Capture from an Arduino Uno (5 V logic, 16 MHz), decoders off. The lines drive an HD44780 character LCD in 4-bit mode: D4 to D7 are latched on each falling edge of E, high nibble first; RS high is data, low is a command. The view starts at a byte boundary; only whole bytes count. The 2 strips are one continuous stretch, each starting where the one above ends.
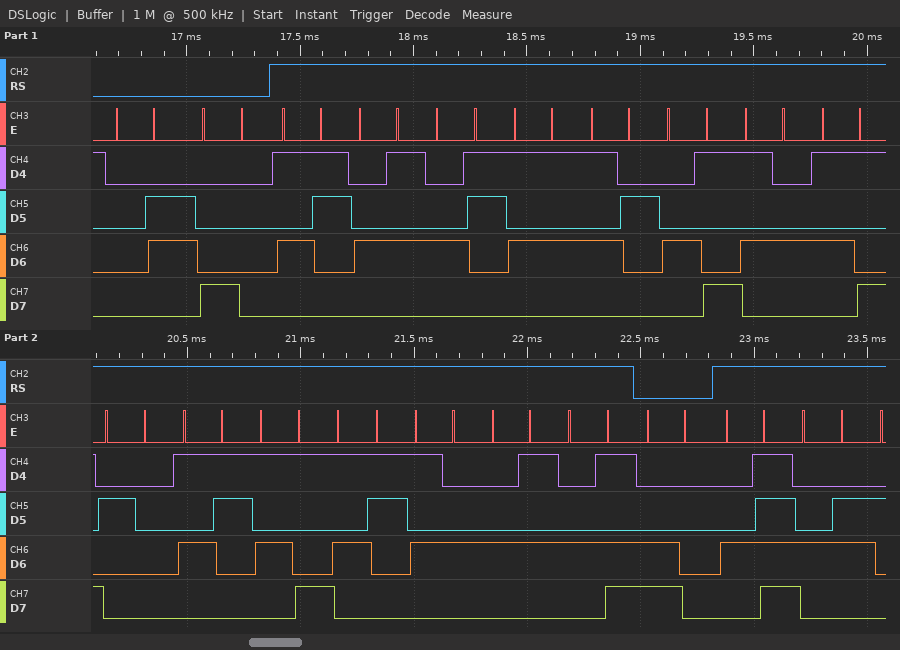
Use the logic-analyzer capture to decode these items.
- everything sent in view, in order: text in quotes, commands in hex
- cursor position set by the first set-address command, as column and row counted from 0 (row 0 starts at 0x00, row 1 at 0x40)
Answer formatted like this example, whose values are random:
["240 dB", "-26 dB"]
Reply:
["0x06 0x80 \"SECURITY SYSTEM\" 0xC0 \"OF\"", "column 0, row 0"]
